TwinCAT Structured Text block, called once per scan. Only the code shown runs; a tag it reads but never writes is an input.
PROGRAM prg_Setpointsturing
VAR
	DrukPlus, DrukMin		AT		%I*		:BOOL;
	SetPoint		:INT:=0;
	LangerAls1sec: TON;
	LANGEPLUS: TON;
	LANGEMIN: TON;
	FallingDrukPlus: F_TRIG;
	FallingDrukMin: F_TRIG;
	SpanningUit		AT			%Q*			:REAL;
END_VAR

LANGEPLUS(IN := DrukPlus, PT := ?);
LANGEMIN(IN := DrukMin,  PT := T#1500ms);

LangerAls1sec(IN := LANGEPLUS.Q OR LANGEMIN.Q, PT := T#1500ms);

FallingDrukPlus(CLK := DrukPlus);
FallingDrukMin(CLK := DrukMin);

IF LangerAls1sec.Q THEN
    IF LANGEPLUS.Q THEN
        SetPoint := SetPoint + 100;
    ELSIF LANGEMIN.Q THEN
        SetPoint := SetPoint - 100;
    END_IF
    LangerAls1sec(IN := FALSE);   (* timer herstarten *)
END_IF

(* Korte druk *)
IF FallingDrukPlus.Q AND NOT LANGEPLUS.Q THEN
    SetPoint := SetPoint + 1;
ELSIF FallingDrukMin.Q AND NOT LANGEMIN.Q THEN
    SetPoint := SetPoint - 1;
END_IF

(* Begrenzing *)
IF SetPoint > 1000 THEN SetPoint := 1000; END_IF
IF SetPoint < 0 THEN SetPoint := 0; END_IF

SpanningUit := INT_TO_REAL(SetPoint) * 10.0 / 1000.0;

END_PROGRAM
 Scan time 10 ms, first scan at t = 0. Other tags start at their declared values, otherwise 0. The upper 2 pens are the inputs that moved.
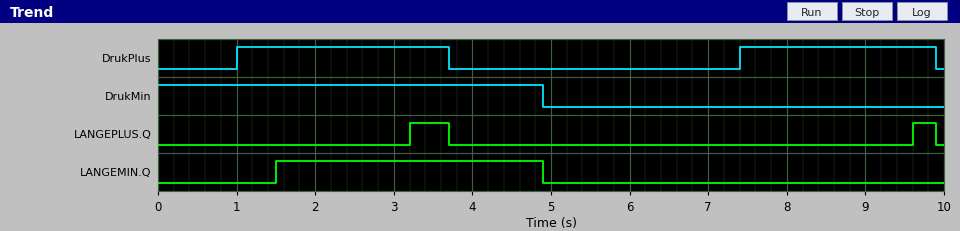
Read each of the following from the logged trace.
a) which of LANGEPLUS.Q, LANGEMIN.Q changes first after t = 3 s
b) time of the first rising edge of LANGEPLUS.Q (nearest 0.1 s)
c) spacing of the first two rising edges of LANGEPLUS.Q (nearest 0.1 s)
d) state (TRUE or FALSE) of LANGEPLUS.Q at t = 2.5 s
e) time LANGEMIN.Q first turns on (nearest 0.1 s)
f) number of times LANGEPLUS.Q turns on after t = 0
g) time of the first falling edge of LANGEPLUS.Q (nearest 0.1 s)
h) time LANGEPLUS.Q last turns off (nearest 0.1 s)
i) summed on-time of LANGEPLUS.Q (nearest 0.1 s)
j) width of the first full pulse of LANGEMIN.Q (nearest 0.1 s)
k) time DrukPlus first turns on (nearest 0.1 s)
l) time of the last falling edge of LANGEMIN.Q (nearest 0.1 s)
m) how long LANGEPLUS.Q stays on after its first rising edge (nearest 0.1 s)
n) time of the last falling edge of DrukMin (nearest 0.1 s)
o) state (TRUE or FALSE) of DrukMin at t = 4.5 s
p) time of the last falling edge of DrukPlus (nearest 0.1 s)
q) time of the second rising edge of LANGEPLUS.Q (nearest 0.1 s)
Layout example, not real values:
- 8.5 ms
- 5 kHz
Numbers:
- LANGEPLUS.Q
- 3.2 s
- 6.4 s
- FALSE
- 1.5 s
- 2
- 3.7 s
- 9.9 s
- 0.8 s
- 3.4 s
- 1.0 s
- 4.9 s
- 0.5 s
- 4.9 s
- TRUE
- 9.9 s
- 9.6 s
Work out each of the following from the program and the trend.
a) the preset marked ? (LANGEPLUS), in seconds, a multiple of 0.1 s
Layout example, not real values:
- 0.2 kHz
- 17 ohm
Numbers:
- 2.2 s
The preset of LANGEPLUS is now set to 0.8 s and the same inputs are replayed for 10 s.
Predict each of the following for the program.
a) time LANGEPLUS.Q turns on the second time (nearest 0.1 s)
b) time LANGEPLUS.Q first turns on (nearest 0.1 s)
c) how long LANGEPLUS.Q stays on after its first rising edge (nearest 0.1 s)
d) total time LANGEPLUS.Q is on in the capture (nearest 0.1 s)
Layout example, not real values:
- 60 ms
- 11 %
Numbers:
- 8.2 s
- 1.8 s
- 1.9 s
- 3.6 s
